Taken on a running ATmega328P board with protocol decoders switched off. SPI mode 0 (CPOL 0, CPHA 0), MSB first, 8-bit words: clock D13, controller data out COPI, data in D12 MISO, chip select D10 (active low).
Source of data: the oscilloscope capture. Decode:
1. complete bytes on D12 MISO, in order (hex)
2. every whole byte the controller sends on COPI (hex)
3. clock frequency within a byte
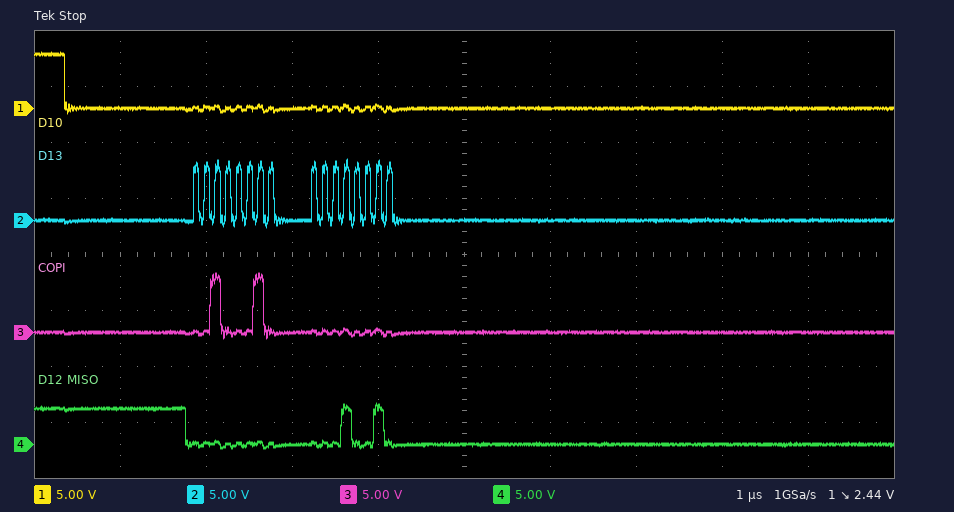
00 12
22 00
8 MHz
